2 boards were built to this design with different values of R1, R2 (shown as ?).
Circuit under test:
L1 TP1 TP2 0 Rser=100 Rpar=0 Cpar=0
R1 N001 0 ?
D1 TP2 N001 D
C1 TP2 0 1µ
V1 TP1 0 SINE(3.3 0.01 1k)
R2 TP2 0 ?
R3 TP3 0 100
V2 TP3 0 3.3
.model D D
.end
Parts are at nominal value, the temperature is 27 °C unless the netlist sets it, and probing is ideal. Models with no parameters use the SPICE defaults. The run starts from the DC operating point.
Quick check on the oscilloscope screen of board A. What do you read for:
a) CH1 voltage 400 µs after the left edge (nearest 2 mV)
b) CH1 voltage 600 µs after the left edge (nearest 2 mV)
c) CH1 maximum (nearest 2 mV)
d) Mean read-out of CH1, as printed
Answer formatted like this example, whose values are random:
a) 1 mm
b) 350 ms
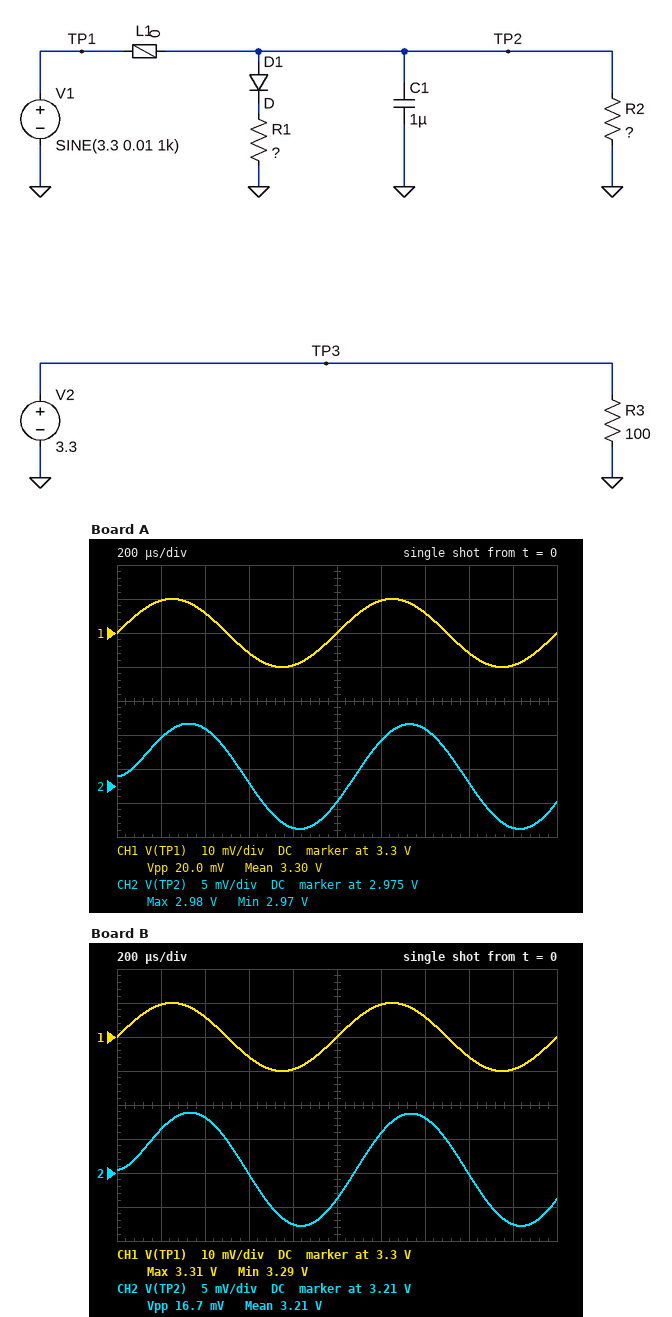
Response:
a) 3.306 V
b) 3.294 V
c) 3.310 V
d) 3.30 V
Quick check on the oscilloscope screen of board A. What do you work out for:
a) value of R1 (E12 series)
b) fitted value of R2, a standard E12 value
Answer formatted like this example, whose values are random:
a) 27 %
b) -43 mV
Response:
a) 820 Ω
b) 6.8 kΩ
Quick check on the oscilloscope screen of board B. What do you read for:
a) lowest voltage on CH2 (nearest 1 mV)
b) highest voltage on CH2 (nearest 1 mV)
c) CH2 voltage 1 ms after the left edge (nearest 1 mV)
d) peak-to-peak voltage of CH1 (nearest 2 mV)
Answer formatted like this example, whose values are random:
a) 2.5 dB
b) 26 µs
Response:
a) 3.202 V
b) 3.219 V
c) 3.206 V
d) 20 mV
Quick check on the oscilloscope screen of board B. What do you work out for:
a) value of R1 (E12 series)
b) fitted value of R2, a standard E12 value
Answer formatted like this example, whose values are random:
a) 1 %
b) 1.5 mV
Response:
a) 3.3 kΩ
b) 27 kΩ
